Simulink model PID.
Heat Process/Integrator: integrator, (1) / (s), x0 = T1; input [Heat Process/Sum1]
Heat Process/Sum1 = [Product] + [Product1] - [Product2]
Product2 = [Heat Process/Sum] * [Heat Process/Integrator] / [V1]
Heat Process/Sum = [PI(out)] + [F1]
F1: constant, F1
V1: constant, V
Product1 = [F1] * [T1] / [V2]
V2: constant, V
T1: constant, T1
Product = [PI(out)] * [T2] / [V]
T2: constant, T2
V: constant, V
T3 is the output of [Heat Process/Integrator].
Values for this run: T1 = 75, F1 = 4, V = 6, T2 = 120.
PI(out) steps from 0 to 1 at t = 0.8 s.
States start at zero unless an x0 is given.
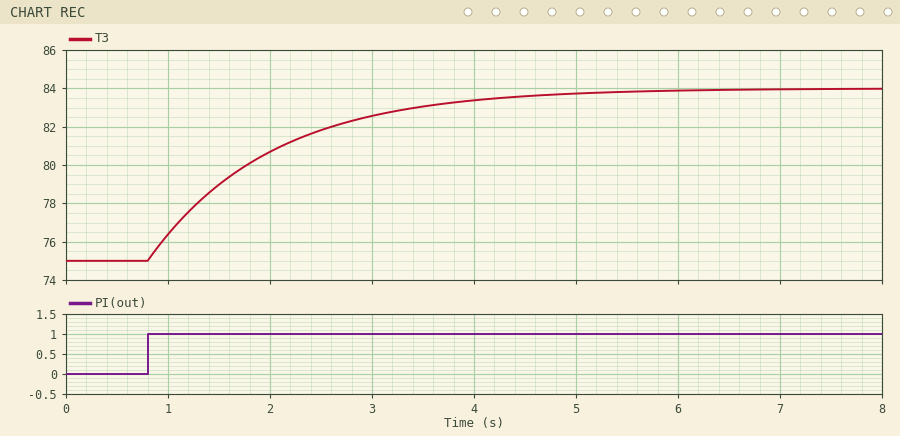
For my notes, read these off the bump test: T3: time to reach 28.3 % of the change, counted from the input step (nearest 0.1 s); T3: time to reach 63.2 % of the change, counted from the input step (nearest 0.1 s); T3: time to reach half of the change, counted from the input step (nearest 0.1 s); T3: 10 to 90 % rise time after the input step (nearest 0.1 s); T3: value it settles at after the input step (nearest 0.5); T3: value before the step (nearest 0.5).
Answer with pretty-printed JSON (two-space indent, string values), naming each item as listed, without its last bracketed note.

{
  "T3: time to reach 28.3 % of the change, counted from the input step": "0.4 s",
  "T3: time to reach 63.2 % of the change, counted from the input step": "1.2 s",
  "T3: time to reach half of the change, counted from the input step": "0.8 s",
  "T3: 10 to 90 % rise time after the input step": "2.6 s",
  "T3: value it settles at after the input step": "84.0",
  "T3: value before the step": "75.0"
}
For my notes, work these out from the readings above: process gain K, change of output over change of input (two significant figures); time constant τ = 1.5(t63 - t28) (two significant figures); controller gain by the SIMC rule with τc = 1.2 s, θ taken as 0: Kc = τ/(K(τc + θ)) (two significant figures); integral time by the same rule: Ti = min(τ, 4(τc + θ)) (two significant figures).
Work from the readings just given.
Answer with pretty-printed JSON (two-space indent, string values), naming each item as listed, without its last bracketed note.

{
  "process gain K, change of output over change of input": "9.0",
  "time constant τ = 1.5(t63 - t28)": "1.2 s",
  "controller gain by the SIMC rule with τc = 1.2 s, θ taken as 0: Kc = τ/(K(τc + θ))": "0.11",
  "integral time by the same rule: Ti = min(τ, 4(τc + θ))": "1.2 s"
}
